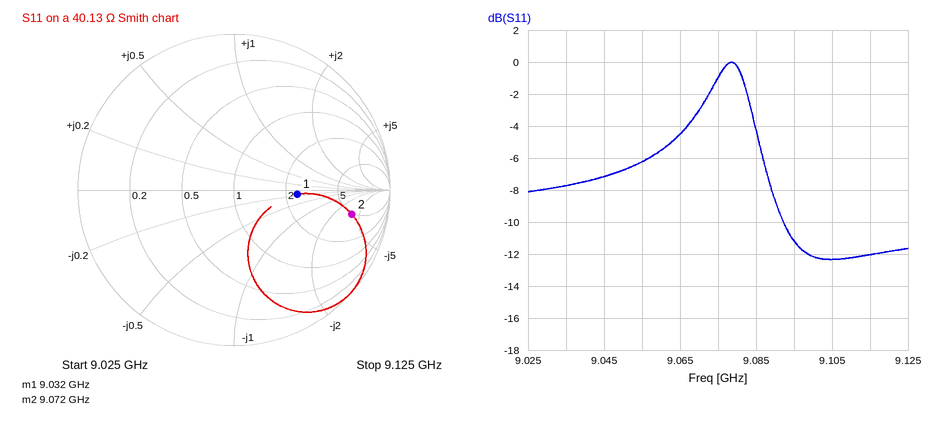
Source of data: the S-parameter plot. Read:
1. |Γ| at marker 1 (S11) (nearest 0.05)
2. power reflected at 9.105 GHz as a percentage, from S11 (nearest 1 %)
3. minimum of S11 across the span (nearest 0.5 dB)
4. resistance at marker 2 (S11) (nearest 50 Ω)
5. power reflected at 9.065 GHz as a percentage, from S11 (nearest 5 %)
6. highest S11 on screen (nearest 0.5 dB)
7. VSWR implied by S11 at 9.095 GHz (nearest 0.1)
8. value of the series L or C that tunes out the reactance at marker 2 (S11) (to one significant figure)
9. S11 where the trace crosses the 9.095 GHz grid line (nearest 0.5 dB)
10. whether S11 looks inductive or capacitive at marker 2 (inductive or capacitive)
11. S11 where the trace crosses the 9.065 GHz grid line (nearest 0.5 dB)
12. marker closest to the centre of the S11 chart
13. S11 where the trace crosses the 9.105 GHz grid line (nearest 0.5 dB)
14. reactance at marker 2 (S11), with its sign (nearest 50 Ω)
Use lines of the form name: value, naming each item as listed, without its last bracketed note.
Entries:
|Γ| at marker 1 (S11): 0.40
power reflected at 9.105 GHz as a percentage, from S11: 6 %
minimum of S11 across the span: -12.5 dB
resistance at marker 2 (S11): 200 Ω
power reflected at 9.065 GHz as a percentage, from S11: 35 %
highest S11 on screen: 0.0 dB
VSWR implied by S11 at 9.095 GHz: 1.8
value of the series L or C that tunes out the reactance at marker 2 (S11): 3 nH
S11 where the trace crosses the 9.095 GHz grid line: -11.0 dB
whether S11 looks inductive or capacitive at marker 2: capacitive
S11 where the trace crosses the 9.065 GHz grid line: -4.5 dB
marker closest to the centre of the S11 chart: marker 1
S11 where the trace crosses the 9.105 GHz grid line: -12.5 dB
reactance at marker 2 (S11), with its sign: -150 Ω
